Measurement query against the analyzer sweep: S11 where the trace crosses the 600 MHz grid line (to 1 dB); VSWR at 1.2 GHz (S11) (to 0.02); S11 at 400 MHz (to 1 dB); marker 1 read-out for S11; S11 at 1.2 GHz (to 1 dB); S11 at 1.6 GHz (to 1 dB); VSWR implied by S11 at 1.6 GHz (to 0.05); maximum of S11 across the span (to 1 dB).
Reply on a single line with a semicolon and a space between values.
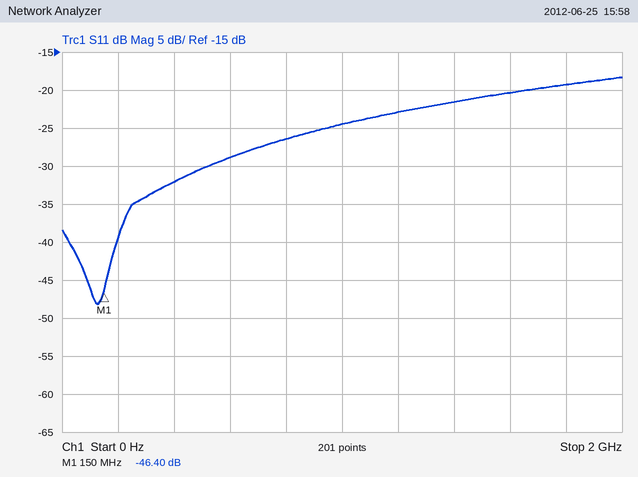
-29 dB; 1.16; -32 dB; -46.40 dB; -23 dB; -20 dB; 1.20; -18 dB
